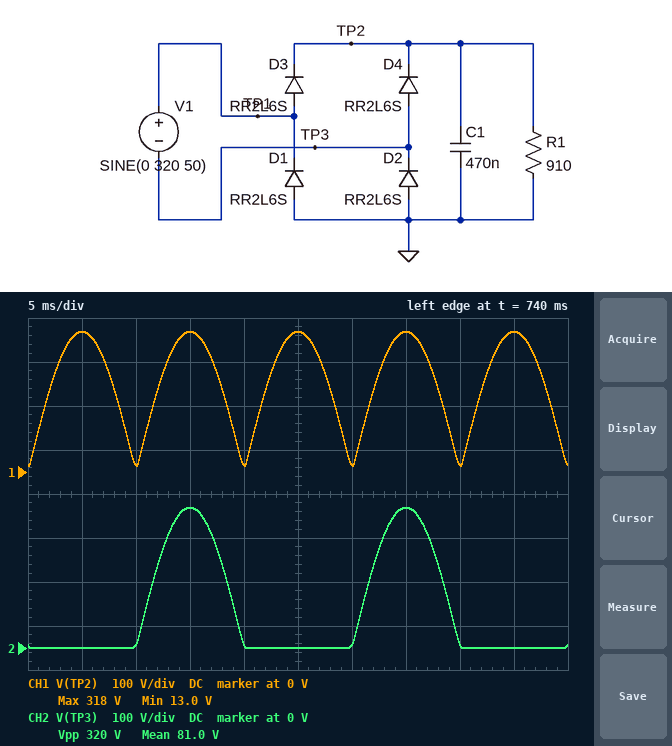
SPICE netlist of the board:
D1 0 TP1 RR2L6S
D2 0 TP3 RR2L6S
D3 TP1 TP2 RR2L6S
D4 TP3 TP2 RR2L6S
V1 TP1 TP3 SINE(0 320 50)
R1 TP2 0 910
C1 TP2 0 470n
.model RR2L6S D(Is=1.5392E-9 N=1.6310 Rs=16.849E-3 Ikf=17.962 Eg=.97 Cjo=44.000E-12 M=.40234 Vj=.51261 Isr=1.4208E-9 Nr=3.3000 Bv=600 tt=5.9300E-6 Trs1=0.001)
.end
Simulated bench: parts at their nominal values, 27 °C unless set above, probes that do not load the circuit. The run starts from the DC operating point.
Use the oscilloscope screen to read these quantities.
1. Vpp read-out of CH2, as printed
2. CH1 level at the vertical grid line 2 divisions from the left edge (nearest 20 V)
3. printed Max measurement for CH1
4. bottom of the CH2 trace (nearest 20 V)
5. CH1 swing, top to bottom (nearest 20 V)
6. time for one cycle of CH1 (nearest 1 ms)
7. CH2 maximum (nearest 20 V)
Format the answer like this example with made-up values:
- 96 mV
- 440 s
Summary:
- 320 V
- 20 V
- 318 V
- 0 V
- 300 V
- 10 ms
- 320 V
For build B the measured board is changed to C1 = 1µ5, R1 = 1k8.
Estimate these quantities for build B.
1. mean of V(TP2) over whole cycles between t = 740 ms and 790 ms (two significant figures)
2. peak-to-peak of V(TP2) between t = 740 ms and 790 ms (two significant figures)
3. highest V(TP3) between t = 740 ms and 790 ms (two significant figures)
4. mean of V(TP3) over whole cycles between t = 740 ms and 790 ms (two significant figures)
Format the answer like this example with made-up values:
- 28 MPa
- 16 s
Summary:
- 210 V
- 250 V
- 320 V
- 110 V
